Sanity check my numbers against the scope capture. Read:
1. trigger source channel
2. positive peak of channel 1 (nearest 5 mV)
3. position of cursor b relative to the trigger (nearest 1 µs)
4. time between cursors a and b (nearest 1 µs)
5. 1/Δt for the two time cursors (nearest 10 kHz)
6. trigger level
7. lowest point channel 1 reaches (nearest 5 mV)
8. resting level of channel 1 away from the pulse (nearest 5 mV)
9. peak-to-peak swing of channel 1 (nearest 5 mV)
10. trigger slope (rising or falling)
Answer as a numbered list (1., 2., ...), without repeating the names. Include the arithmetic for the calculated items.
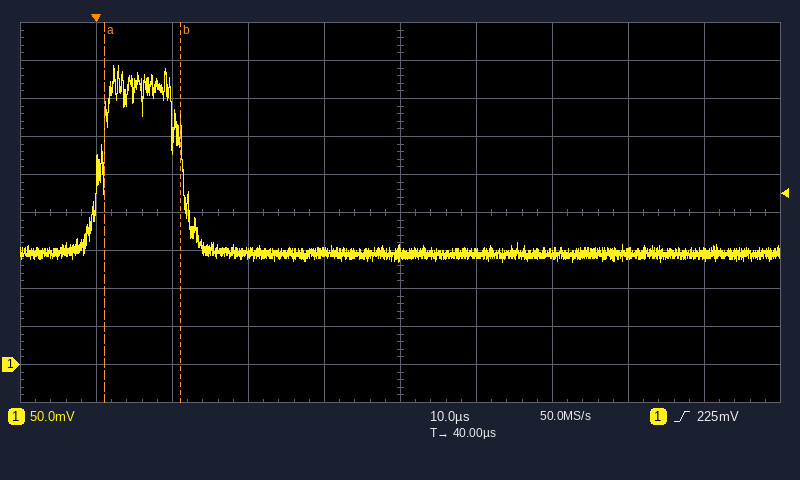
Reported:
1. channel 1
2. 395 mV
3. +11 µs
4. 10 µs
5. 1 / 10 µs ≈ 100 kHz
6. 225 mV
7. 135 mV
8. 145 mV
9. 395 mV − (135 mV) = 260 mV
10. rising
